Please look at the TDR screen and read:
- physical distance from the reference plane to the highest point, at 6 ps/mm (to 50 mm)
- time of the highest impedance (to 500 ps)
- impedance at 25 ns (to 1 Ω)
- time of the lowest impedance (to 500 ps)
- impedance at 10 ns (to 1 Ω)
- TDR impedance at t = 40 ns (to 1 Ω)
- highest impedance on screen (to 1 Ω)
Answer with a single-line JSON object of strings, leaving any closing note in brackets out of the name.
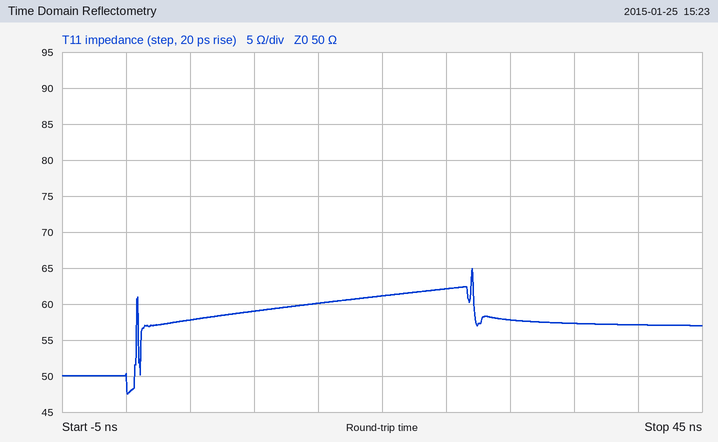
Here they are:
{"physical distance from the reference plane to the highest point, at 6 ps/mm": "2.25 m", "time of the highest impedance": "27.0 ns", "impedance at 25 ns": "62 Ω", "time of the lowest impedance": "0.0 ns", "impedance at 10 ns": "59 Ω", "TDR impedance at t = 40 ns": "57 Ω", "highest impedance on screen": "65 Ω"}
